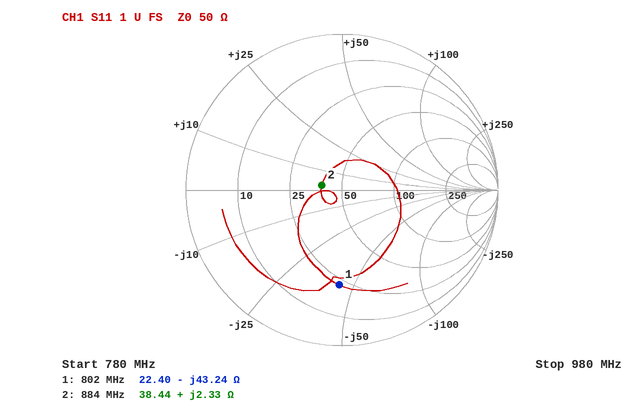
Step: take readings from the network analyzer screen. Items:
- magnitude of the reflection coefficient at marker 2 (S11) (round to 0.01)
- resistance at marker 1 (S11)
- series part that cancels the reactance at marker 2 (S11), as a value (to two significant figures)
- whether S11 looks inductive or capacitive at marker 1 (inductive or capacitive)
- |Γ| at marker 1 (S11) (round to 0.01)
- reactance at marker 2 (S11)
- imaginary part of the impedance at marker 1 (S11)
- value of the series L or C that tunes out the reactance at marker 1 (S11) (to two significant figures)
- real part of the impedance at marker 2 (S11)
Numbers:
0.13
22.40 Ω
77 pF
capacitive
0.61
+2.33 Ω
-43.24 Ω
8.6 nH
38.44 Ω
